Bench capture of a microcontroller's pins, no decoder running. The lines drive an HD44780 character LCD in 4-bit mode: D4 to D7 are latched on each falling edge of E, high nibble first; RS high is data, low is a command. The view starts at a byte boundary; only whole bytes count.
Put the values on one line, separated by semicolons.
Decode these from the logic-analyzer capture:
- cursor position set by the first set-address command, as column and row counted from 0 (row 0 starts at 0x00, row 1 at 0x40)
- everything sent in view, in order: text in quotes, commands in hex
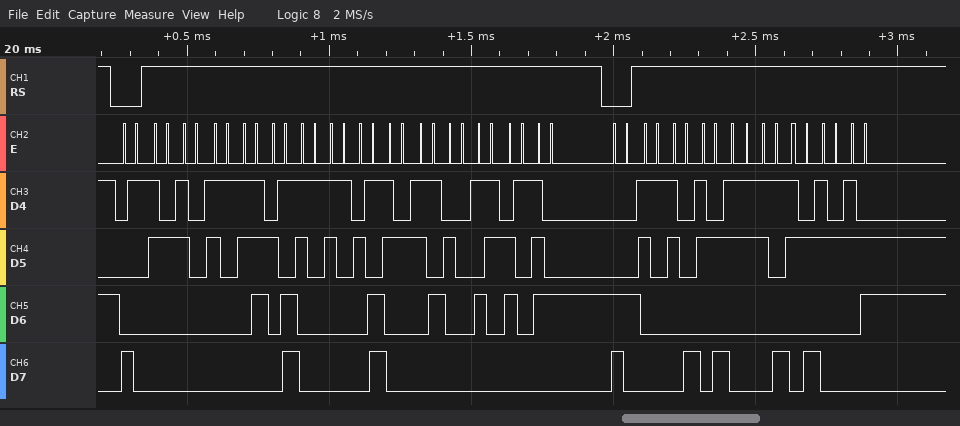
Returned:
column 1, row 0; 0x81 "2017-11-25 Sat" 0xC4 "18:39:26"
